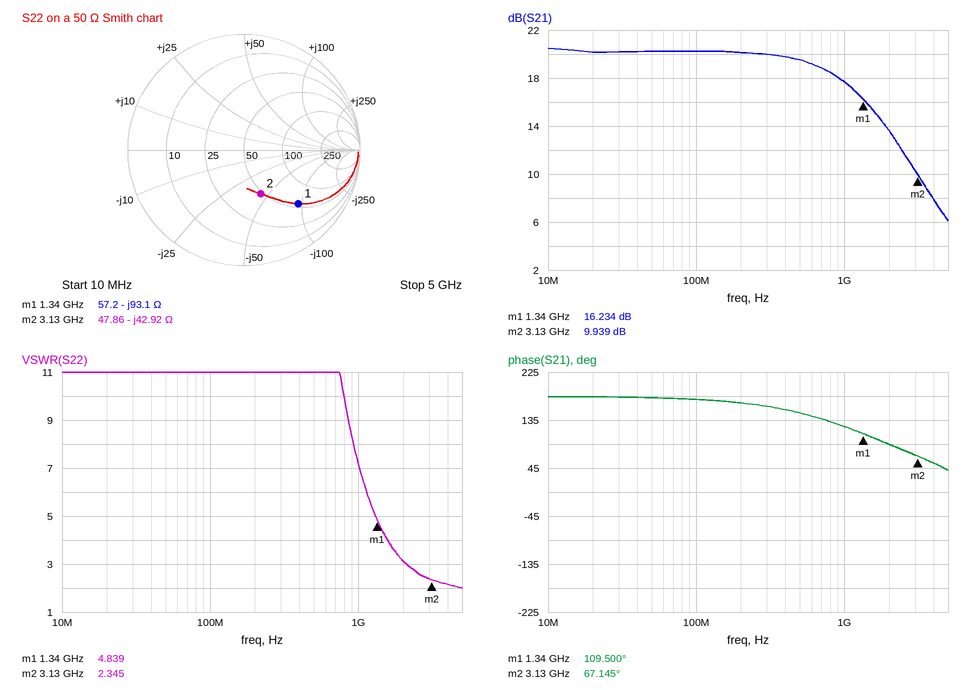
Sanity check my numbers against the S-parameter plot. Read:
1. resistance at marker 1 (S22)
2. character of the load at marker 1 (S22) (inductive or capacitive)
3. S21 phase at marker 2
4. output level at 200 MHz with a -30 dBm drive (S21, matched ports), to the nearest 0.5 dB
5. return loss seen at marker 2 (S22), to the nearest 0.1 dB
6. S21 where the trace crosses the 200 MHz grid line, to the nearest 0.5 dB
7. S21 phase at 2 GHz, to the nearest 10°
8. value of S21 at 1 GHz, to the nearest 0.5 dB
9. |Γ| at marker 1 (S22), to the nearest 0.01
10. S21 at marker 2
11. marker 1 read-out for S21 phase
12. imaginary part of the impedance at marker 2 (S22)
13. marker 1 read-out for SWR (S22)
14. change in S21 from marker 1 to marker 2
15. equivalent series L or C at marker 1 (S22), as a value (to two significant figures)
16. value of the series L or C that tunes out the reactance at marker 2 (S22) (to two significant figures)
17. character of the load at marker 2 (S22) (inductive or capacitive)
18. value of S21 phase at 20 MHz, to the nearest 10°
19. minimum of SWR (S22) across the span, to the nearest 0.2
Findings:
57.2 Ω
capacitive
67.145°
-10.0 dBm
7.9 dB
20.0 dB
90°
17.5 dB
0.66
9.939 dB
109.500°
-42.92 Ω
4.839
-6.295 dB
1.3 pF
2.2 nH
capacitive
180°
2.0
